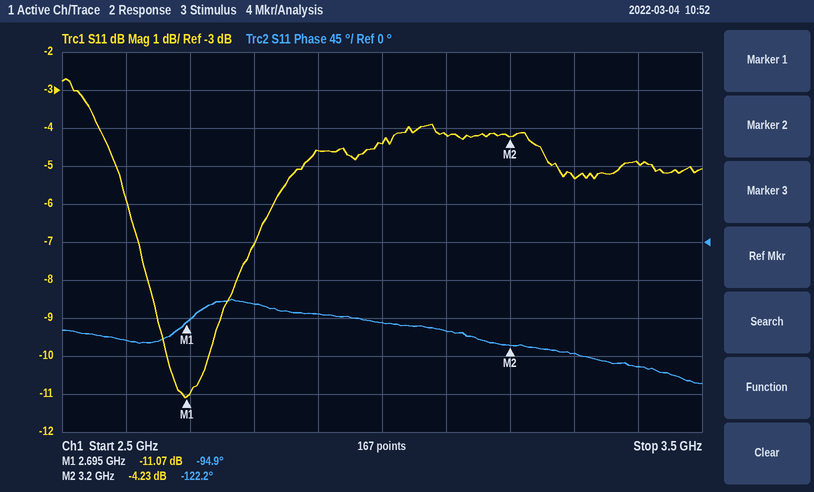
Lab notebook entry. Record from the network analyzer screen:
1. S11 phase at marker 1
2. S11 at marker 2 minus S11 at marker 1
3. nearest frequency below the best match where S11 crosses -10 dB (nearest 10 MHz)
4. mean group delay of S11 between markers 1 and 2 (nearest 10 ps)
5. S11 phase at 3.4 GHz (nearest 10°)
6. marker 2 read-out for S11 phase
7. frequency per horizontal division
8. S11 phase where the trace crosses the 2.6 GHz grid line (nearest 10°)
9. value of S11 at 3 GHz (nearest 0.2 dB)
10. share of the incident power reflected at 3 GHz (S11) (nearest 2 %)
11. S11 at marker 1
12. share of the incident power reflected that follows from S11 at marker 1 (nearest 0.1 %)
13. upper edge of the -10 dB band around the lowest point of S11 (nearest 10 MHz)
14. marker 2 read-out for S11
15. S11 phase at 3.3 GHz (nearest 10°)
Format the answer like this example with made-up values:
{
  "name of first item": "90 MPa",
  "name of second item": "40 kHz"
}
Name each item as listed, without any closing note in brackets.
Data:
{
  "S11 phase at marker 1": "-94.9°",
  "S11 at marker 2 minus S11 at marker 1": "6.84 dB",
  "nearest frequency below the best match where S11 crosses -10 dB": "2.66 GHz",
  "mean group delay of S11 between markers 1 and 2": "150 ps",
  "S11 phase at 3.4 GHz": "-150°",
  "marker 2 read-out for S11 phase": "-122.2°",
  "frequency per horizontal division": "100 MHz",
  "S11 phase where the trace crosses the 2.6 GHz grid line": "-120°",
  "value of S11 at 3 GHz": "-4.4 dB",
  "share of the incident power reflected at 3 GHz (S11)": "36 %",
  "S11 at marker 1": "-11.07 dB",
  "share of the incident power reflected that follows from S11 at marker 1": "7.8 %",
  "upper edge of the -10 dB band around the lowest point of S11": "2.73 GHz",
  "marker 2 read-out for S11": "-4.23 dB",
  "S11 phase at 3.3 GHz": "-130°"
}
